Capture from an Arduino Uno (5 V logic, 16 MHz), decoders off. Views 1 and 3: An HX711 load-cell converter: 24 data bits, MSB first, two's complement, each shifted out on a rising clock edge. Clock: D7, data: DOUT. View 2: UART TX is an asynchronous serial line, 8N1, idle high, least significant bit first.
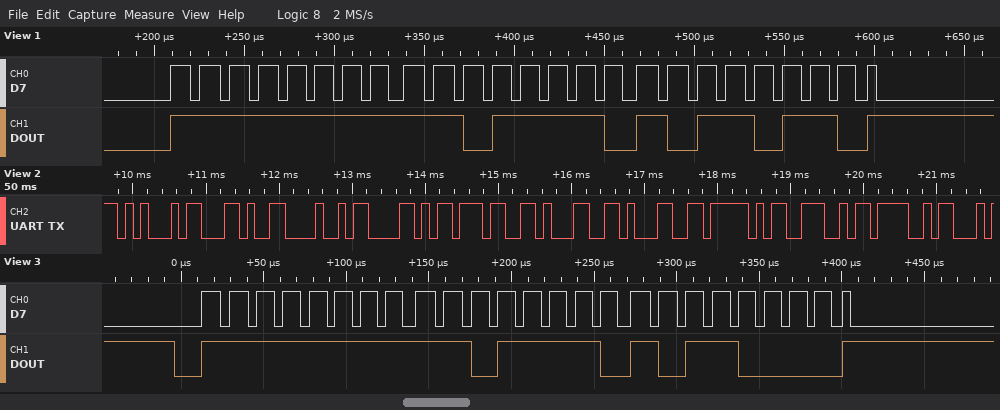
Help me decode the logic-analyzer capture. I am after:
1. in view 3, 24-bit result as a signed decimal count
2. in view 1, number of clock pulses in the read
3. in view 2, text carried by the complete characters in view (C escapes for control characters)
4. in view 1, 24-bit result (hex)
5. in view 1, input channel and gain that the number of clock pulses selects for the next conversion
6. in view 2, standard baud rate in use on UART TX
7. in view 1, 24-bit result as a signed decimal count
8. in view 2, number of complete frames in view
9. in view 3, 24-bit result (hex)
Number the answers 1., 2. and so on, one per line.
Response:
1. -8528
2. 25
3. "E,HX711_NO"
4. 0xFFDEB6
5. channel A, gain 128
6. 9600 baud
7. -8522
8. 10
9. 0xFFDEB0
